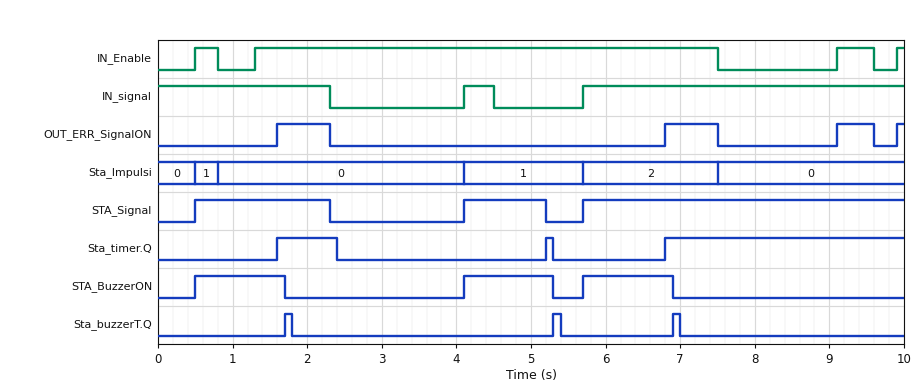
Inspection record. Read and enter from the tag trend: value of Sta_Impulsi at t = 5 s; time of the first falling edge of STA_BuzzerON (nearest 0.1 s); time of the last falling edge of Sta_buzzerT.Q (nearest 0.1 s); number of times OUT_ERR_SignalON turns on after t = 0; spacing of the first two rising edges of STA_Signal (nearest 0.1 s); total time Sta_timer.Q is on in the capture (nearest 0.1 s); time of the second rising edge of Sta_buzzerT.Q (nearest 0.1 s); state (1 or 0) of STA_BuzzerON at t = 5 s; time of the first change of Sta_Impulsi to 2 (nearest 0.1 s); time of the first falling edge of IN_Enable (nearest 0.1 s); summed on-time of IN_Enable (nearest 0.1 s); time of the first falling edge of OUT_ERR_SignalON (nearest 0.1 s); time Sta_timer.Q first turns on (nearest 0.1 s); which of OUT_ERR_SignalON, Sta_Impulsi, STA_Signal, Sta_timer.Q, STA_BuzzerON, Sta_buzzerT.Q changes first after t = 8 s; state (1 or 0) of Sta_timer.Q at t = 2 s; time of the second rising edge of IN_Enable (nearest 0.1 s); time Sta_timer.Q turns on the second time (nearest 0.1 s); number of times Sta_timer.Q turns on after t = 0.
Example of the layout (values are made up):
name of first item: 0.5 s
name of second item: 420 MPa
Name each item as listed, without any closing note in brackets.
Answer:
value of Sta_Impulsi at t = 5 s: 1
time of the first falling edge of STA_BuzzerON: 1.7 s
time of the last falling edge of Sta_buzzerT.Q: 7.0 s
number of times OUT_ERR_SignalON turns on after t = 0: 4
spacing of the first two rising edges of STA_Signal: 3.6 s
total time Sta_timer.Q is on in the capture: 4.1 s
time of the second rising edge of Sta_buzzerT.Q: 5.3 s
state (1 or 0) of STA_BuzzerON at t = 5 s: 1
time of the first change of Sta_Impulsi to 2: 5.7 s
time of the first falling edge of IN_Enable: 0.8 s
summed on-time of IN_Enable: 7.1 s
time of the first falling edge of OUT_ERR_SignalON: 2.3 s
time Sta_timer.Q first turns on: 1.6 s
which of OUT_ERR_SignalON, Sta_Impulsi, STA_Signal, Sta_timer.Q, STA_BuzzerON, Sta_buzzerT.Q changes first after t = 8 s: OUT_ERR_SignalON
state (1 or 0) of Sta_timer.Q at t = 2 s: 1
time of the second rising edge of IN_Enable: 1.3 s
time Sta_timer.Q turns on the second time: 5.2 s
number of times Sta_timer.Q turns on after t = 0: 3
